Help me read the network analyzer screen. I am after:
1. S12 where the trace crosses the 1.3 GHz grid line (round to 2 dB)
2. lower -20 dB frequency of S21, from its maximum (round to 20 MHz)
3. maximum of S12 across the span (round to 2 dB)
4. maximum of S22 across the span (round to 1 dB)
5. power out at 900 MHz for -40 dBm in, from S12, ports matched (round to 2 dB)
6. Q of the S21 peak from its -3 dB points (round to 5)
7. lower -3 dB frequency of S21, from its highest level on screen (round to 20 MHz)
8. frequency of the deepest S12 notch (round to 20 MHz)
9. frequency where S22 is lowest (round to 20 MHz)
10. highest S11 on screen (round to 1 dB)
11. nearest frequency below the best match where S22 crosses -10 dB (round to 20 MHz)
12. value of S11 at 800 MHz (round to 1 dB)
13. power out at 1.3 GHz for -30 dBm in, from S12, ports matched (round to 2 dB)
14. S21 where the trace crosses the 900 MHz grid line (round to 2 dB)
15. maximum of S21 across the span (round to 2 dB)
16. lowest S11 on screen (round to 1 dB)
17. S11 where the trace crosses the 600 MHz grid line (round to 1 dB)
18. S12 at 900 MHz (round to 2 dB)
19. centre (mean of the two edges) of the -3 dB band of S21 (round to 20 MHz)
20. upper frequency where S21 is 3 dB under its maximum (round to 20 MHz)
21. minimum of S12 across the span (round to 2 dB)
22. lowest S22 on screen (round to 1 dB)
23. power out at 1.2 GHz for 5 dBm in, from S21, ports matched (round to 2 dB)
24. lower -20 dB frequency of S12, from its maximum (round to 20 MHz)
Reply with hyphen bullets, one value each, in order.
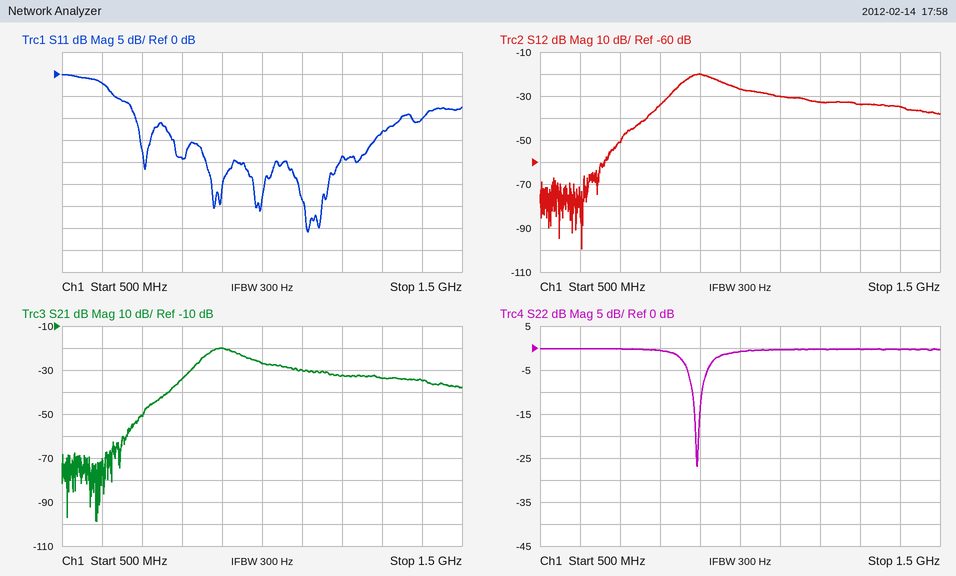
- -34 dB
- 760 MHz
- -20 dB
- 0 dB
- -60 dBm
- 10
- 860 MHz
- 600 MHz
- 900 MHz
- 0 dB
- 880 MHz
- -19 dB
- -64 dBm
- -20 dB
- -20 dB
- -36 dB
- -2 dB
- -20 dB
- 900 MHz
- 940 MHz
- -100 dB
- -27 dB
- -28 dBm
- 760 MHz
